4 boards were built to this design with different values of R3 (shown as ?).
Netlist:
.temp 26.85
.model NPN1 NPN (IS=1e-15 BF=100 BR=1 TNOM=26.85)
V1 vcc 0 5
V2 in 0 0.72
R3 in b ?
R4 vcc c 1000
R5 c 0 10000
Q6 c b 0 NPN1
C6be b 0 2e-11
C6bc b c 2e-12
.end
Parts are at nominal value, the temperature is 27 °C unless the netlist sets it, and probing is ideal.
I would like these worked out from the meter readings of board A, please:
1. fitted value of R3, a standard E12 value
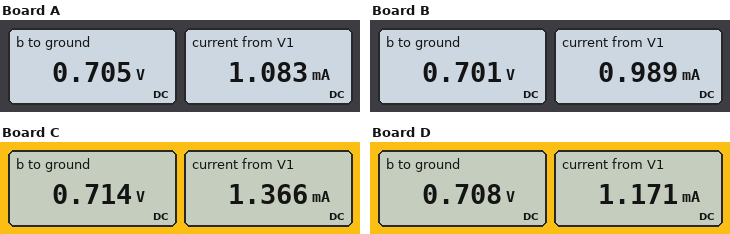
2.2 kΩ
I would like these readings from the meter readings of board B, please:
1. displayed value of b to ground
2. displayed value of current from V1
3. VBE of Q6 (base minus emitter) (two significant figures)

0.701 V
0.989 mA
700 mV
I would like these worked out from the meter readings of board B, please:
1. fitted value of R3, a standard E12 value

3.3 kΩ
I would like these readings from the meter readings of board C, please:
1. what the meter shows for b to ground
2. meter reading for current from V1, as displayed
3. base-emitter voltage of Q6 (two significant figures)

0.714 V
1.366 mA
710 mV
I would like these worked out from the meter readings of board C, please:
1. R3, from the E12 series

560 Ω
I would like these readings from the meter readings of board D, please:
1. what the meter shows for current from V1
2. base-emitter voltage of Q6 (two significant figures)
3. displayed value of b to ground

1.171 mA
710 mV
0.708 V
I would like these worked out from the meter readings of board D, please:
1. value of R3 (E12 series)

1.5 kΩ
